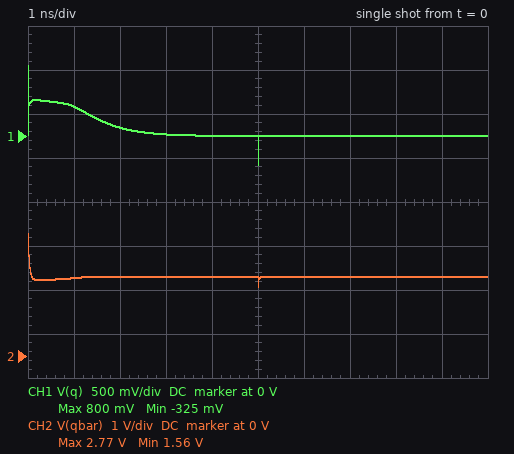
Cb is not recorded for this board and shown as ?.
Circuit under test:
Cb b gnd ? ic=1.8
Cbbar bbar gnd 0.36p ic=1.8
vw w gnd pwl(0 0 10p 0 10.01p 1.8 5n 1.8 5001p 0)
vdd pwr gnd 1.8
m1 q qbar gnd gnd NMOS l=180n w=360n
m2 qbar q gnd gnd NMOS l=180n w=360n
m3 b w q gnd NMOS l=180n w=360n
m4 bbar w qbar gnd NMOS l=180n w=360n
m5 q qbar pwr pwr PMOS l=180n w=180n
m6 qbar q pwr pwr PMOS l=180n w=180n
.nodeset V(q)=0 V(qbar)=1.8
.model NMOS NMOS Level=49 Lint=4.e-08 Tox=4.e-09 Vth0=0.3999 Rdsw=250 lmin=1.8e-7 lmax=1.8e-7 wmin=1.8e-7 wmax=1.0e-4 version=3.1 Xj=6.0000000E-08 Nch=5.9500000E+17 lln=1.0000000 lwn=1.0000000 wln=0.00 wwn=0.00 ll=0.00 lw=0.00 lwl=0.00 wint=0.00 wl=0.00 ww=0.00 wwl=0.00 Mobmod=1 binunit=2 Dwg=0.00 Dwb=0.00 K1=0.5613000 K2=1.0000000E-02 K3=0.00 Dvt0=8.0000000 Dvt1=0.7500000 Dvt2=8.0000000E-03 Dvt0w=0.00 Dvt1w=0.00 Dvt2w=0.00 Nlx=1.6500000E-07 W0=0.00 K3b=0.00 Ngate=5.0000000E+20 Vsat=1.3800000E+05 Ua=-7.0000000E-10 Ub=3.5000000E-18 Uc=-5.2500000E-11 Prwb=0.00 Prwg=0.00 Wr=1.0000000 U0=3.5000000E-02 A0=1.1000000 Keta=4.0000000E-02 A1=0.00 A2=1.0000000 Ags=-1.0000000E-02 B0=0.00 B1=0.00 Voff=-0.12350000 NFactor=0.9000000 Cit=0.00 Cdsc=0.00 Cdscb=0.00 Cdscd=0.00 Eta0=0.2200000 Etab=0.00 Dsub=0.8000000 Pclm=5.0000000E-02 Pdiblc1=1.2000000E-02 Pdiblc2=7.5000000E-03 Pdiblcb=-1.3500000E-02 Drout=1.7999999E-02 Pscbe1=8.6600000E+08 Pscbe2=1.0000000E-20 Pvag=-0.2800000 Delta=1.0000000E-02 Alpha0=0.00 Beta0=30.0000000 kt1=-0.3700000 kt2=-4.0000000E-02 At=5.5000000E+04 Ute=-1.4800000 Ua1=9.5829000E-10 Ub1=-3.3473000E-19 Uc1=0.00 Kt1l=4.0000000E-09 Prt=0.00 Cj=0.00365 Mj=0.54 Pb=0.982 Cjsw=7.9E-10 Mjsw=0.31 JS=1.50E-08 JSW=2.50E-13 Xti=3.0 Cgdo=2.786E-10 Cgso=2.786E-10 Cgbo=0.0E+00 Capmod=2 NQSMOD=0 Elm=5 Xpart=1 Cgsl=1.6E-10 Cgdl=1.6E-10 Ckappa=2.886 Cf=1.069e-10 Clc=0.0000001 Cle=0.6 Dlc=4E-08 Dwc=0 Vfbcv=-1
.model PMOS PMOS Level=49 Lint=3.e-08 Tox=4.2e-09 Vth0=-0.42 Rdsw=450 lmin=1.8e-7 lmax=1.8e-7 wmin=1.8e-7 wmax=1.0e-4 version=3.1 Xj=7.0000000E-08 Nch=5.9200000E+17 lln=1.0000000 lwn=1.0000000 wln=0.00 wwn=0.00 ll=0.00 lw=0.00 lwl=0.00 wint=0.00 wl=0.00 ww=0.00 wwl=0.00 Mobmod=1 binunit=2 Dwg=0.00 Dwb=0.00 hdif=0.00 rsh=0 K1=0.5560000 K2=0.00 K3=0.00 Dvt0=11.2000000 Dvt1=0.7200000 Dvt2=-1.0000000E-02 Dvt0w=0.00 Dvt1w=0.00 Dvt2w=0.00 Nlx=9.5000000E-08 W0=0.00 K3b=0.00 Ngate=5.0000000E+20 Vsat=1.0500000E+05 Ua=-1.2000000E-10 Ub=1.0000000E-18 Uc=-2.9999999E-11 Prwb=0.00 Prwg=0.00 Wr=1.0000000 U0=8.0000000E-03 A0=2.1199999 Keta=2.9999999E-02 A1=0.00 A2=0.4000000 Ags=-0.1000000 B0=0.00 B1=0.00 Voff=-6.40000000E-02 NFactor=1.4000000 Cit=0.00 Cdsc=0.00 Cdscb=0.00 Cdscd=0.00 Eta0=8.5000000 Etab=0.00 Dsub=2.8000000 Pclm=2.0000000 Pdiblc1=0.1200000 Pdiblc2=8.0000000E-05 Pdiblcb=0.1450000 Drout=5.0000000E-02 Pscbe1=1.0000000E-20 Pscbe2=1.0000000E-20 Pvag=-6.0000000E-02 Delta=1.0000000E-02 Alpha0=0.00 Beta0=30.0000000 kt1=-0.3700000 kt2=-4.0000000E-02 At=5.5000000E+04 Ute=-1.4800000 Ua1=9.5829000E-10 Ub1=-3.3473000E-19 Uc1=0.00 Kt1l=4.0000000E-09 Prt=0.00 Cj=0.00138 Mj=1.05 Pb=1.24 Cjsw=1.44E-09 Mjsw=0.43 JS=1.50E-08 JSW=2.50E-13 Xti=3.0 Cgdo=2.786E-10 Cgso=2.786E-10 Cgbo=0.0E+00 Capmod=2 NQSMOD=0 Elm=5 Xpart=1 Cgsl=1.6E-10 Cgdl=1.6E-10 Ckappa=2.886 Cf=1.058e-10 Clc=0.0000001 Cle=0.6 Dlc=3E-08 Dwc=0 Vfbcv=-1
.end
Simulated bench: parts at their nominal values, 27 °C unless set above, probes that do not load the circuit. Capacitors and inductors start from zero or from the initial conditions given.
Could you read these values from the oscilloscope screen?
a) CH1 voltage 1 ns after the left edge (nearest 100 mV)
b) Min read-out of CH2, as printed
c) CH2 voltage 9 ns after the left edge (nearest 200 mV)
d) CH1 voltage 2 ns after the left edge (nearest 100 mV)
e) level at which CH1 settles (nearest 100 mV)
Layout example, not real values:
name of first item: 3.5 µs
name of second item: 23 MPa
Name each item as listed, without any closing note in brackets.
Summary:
CH1 voltage 1 ns after the left edge: 300 mV
Min read-out of CH2, as printed: 1.56 V
CH2 voltage 9 ns after the left edge: 1.8 V
CH1 voltage 2 ns after the left edge: 100 mV
level at which CH1 settles: 0 V
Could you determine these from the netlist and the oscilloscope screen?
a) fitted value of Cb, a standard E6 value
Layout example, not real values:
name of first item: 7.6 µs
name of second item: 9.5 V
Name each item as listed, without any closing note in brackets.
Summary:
fitted value of Cb, a standard E6 value: 150 fF
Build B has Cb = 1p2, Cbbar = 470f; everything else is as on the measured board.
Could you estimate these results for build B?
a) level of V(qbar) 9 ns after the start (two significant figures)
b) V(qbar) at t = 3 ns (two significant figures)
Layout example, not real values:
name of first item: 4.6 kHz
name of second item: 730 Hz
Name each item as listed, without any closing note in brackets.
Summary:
level of V(qbar) 9 ns after the start: 1.8 V
V(qbar) at t = 3 ns: 1.7 V
